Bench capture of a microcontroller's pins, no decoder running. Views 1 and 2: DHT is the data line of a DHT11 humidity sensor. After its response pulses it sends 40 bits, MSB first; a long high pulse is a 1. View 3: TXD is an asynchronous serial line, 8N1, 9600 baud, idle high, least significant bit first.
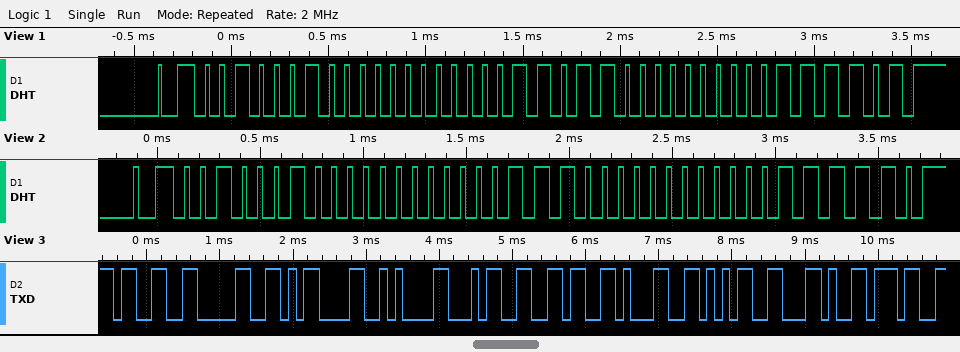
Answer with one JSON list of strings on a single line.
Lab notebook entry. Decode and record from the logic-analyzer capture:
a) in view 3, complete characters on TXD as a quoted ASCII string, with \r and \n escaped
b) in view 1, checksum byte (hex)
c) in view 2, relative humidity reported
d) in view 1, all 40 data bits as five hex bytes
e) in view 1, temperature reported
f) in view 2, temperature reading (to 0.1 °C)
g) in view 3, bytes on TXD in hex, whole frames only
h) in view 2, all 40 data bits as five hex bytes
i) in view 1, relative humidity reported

["\"30\\r\\n4615,7\"", "0x3D", "34 %", "22 00 1B 00 3D", "27.0 °C", "28.0 °C", "0x33 0x30 0x0D 0x0A 0x34 0x36 0x31 0x35 0x2C 0x37", "22 00 1C 00 3E", "34 %"]
